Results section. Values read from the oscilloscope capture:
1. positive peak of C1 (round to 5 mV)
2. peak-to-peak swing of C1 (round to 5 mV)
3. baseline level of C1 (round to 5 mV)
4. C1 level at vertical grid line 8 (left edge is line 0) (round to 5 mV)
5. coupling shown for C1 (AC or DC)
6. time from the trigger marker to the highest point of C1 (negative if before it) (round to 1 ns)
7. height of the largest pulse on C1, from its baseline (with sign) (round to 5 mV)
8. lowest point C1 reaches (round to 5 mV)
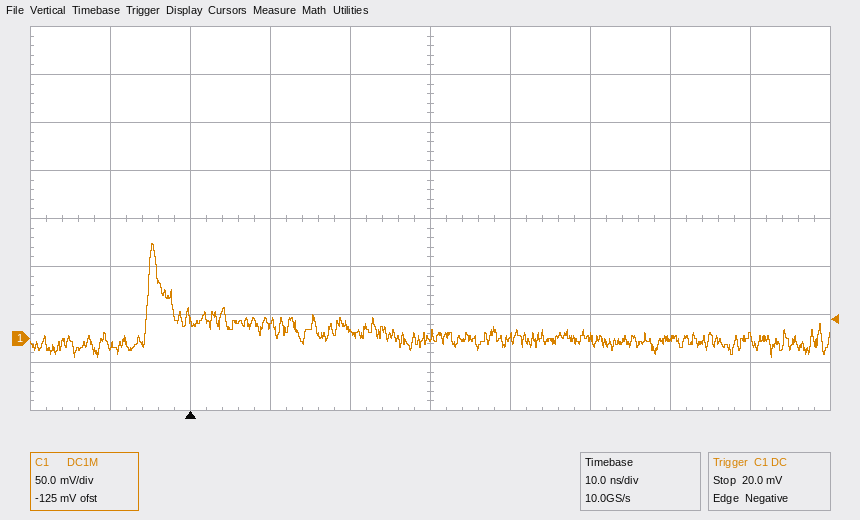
100 mV
120 mV
0 mV
0 mV
DC
-5 ns
+100 mV
-20 mV
